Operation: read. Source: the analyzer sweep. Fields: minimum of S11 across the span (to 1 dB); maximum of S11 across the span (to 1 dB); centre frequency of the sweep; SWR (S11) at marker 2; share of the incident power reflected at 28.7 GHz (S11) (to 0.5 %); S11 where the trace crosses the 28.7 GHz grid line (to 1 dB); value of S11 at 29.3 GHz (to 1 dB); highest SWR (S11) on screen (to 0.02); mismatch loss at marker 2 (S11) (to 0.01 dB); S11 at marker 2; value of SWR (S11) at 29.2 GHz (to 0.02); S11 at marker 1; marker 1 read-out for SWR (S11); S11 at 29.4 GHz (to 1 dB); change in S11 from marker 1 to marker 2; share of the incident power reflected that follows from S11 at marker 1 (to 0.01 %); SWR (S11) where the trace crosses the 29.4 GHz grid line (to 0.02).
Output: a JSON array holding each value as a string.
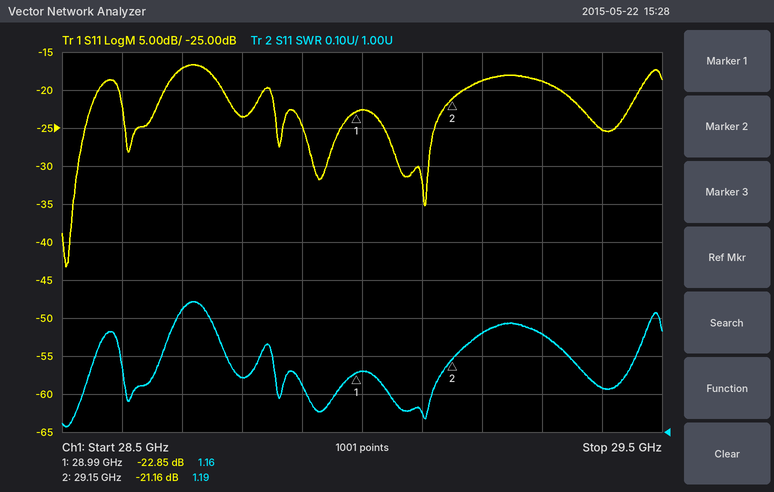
["-43 dB", "-17 dB", "29 GHz", "1.19", "2.0 %", "-17 dB", "-19 dB", "1.34", "0.03 dB", "-21.16 dB", "1.26", "-22.85 dB", "1.16", "-25 dB", "1.69 dB", "0.52 %", "1.12"]
